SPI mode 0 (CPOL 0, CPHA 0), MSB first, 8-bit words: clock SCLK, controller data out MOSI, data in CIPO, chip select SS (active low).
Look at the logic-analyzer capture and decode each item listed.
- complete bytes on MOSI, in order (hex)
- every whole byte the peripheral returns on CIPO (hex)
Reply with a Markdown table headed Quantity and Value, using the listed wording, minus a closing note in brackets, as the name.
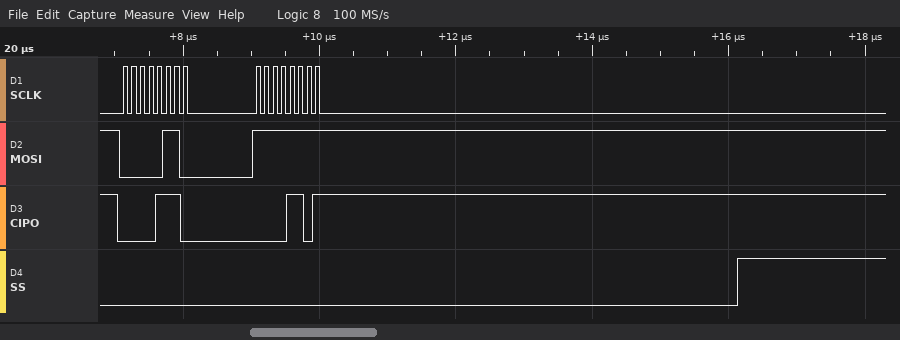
| Quantity | Value |
|---|---|
| complete bytes on MOSI, in order | 06 FF |
| every whole byte the peripheral returns on CIPO | 0E 0D |
